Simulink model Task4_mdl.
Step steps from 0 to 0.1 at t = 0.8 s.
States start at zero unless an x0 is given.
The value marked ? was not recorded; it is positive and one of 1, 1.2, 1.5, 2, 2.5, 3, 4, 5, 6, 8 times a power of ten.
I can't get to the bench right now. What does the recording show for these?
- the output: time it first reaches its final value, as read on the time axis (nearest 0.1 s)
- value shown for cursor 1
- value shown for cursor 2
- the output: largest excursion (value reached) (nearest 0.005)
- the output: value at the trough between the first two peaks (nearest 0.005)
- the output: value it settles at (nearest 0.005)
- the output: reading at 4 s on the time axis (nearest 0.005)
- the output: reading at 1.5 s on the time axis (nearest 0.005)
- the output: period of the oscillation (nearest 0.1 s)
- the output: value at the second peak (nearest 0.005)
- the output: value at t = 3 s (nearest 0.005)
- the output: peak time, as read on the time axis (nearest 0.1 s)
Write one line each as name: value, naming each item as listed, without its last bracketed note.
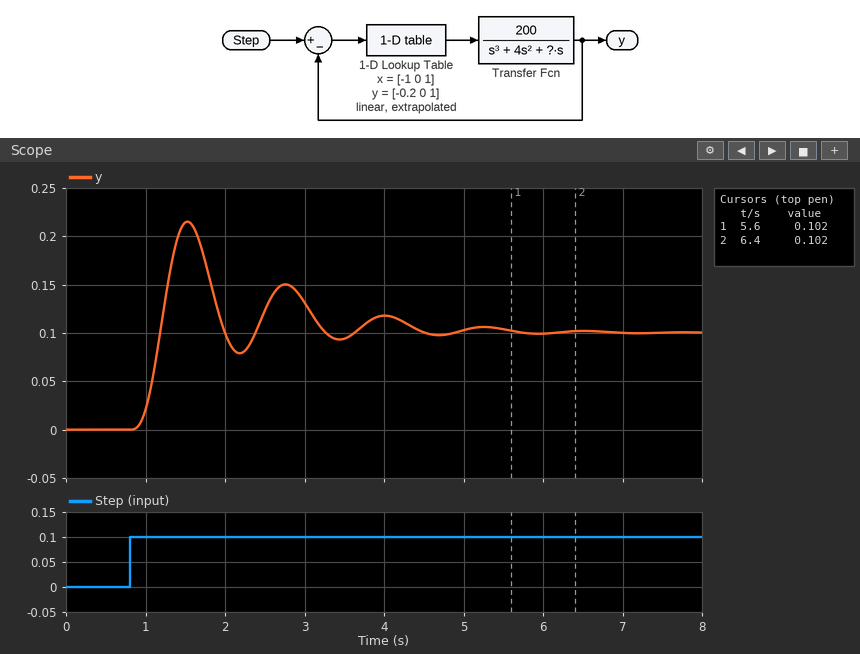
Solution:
the output: time it first reaches its final value, as read on the time axis: 1.2 s
value shown for cursor 1: 0.102
value shown for cursor 2: 0.102
the output: largest excursion (value reached): 0.215
the output: value at the trough between the first two peaks: 0.080
the output: value it settles at: 0.100
the output: reading at 4 s on the time axis: 0.120
the output: reading at 1.5 s on the time axis: 0.215
the output: period of the oscillation: 1.2 s
the output: value at the second peak: 0.150
the output: value at t = 3 s: 0.130
the output: peak time, as read on the time axis: 1.5 s
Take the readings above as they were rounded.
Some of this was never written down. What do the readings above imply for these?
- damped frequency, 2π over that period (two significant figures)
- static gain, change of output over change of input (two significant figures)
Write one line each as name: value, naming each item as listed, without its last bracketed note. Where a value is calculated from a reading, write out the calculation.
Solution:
damped frequency, 2π over that period: 2π / 1.2 = 5.2 rad/s
static gain, change of output over change of input: (0.1 - 0) / (0.1 - 0) = 1.0
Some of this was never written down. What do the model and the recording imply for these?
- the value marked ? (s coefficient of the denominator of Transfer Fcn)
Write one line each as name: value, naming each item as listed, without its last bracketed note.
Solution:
the value marked ?: 30
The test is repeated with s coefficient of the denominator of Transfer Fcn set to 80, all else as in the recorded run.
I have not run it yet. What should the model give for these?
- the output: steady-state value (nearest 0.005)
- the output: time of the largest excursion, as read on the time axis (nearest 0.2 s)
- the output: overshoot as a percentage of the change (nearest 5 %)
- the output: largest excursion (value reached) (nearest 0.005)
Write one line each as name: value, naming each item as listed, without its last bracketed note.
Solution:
the output: steady-state value: 0.100
the output: time of the largest excursion, as read on the time axis: 2.0 s
the output: overshoot as a percentage of the change: 10 %
the output: largest excursion (value reached): 0.110
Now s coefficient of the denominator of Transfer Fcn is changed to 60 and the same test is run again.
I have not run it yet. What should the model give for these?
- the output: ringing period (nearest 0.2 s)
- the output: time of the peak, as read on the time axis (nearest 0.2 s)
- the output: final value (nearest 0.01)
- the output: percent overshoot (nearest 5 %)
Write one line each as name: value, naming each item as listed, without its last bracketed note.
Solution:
the output: ringing period: 0.8 s
the output: time of the peak, as read on the time axis: 1.4 s
the output: final value: 0.10
the output: percent overshoot: 25 %
